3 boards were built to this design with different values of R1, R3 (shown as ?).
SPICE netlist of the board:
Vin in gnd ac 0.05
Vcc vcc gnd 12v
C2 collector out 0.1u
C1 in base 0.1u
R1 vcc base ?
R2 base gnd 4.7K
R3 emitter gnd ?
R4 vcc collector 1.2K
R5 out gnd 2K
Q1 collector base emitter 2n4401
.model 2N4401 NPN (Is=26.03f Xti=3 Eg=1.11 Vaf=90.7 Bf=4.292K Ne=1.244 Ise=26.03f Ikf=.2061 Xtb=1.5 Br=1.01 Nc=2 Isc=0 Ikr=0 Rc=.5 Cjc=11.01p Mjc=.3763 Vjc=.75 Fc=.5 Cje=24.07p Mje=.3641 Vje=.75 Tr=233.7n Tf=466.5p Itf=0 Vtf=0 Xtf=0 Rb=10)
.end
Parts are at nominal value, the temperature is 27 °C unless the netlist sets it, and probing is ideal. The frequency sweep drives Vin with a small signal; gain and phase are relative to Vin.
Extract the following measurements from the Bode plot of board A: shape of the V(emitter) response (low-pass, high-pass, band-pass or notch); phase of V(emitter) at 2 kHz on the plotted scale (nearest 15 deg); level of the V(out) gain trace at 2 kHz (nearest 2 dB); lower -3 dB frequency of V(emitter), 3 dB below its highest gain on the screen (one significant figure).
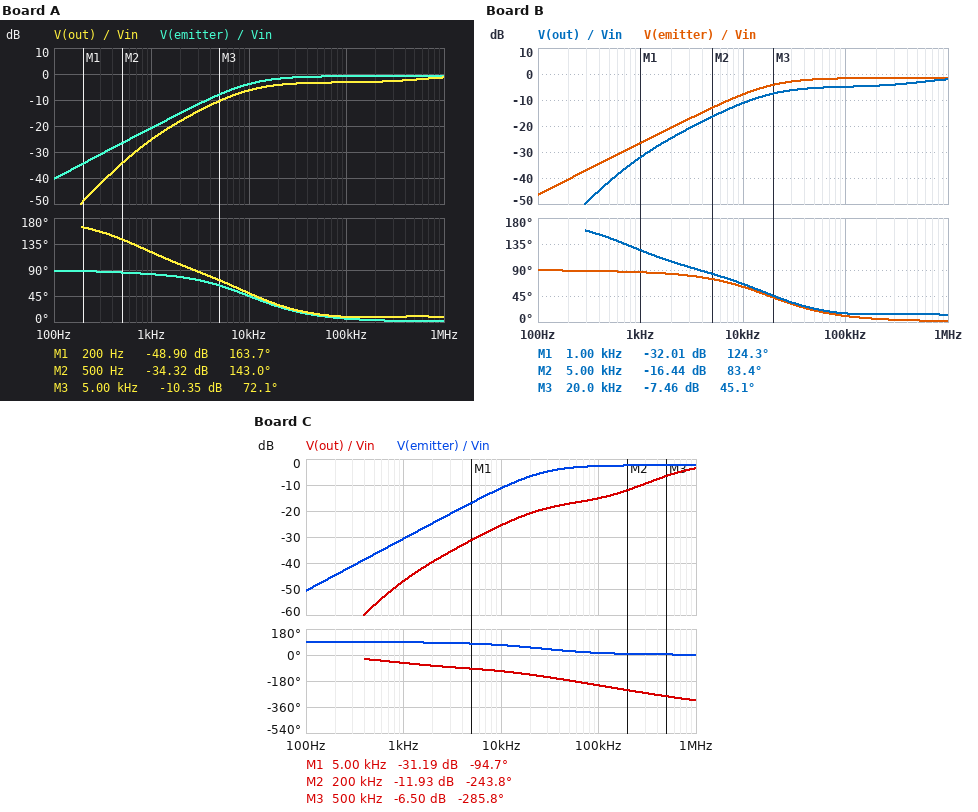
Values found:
high-pass
75 deg
-18 dB
10 kHz
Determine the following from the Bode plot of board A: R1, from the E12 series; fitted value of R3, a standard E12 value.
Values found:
8.2 kΩ
180 Ω
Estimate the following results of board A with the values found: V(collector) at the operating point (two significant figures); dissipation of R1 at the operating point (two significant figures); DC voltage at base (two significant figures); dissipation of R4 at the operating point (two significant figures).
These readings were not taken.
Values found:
1.7 V
11 mW
2.4 V
88 mW
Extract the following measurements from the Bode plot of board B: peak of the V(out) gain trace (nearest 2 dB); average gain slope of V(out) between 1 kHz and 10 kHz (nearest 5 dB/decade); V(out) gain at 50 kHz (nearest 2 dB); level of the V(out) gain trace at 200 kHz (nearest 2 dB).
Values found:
-2 dB
20 dB/decade
-6 dB
-4 dB
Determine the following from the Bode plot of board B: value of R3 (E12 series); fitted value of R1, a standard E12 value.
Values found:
82 Ω
8.2 kΩ
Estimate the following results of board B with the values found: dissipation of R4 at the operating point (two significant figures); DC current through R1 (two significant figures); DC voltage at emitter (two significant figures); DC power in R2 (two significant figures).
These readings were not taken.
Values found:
100 mW
1.3 mA
840 mV
500 µW
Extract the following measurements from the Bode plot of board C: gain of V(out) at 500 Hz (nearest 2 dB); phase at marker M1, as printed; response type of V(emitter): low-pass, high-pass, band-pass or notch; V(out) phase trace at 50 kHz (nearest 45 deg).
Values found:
-56 dB
-94.7 deg
high-pass
-180 deg
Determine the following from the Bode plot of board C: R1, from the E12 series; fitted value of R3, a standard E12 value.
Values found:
15 kΩ
47 Ω
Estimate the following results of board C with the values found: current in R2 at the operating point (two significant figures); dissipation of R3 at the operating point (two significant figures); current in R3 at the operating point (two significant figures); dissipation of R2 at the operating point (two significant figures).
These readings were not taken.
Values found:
250 µA
4.7 mW
10 mA
290 µW
